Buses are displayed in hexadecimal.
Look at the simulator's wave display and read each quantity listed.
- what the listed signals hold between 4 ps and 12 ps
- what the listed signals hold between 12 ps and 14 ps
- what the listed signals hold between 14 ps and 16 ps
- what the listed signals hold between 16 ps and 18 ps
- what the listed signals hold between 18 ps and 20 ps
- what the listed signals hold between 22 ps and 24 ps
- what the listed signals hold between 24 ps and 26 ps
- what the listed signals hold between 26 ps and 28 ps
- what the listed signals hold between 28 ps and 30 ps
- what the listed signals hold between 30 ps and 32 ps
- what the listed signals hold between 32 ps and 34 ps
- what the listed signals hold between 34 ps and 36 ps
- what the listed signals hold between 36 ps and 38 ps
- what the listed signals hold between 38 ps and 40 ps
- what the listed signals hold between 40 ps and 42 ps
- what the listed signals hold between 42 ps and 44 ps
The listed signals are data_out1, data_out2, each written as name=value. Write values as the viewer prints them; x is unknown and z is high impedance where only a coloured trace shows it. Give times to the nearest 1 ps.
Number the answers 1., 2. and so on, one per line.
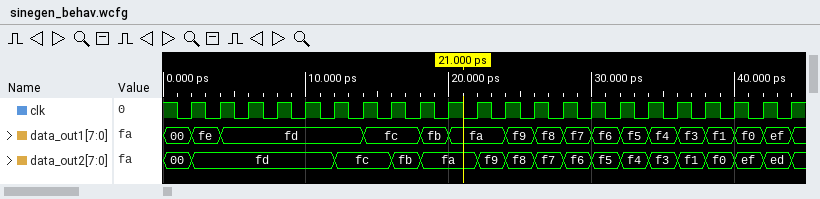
1. data_out1=fd, data_out2=fd
2. data_out1=fd, data_out2=fc
3. data_out1=fc, data_out2=fc
4. data_out1=fc, data_out2=fb
5. data_out1=fb, data_out2=fa
6. data_out1=fa, data_out2=f9
7. data_out1=f9, data_out2=f8
8. data_out1=f8, data_out2=f7
9. data_out1=f7, data_out2=f6
10. data_out1=f6, data_out2=f5
11. data_out1=f5, data_out2=f4
12. data_out1=f4, data_out2=f3
13. data_out1=f3, data_out2=f1
14. data_out1=f1, data_out2=f0
15. data_out1=f0, data_out2=ef
16. data_out1=ef, data_out2=ed
